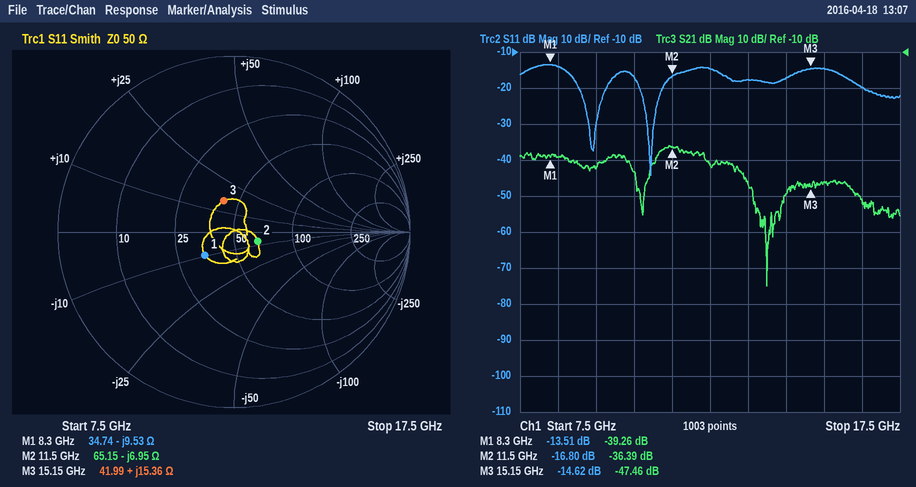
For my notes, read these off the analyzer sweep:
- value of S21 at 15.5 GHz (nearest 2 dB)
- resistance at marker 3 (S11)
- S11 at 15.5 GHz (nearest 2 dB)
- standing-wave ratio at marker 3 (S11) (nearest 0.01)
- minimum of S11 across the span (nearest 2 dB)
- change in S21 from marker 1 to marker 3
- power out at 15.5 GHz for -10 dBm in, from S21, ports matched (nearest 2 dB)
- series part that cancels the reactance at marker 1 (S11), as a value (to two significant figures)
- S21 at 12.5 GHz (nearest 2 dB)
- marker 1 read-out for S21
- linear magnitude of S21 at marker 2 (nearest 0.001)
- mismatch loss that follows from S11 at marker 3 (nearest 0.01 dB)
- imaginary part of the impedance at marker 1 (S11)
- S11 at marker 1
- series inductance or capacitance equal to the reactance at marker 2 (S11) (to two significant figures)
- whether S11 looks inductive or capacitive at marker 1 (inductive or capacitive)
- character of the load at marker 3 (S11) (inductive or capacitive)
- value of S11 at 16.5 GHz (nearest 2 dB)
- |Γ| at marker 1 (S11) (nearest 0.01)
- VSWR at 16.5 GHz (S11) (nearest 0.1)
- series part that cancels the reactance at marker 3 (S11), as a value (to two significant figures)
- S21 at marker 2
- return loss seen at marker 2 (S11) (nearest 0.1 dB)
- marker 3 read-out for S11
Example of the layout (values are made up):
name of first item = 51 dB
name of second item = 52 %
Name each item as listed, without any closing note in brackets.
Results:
value of S21 at 15.5 GHz = -46 dB
resistance at marker 3 = 41.99 Ω
S11 at 15.5 GHz = -14 dB
standing-wave ratio at marker 3 (S11) = 1.46
minimum of S11 across the span = -44 dB
change in S21 from marker 1 to marker 3 = -8.20 dB
power out at 15.5 GHz for -10 dBm in, from S21, ports matched = -56 dBm
series part that cancels the reactance at marker 1 (S11), as a value = 180 pH
S21 at 12.5 GHz = -42 dB
marker 1 read-out for S21 = -39.26 dB
linear magnitude of S21 at marker 2 = 0.015
mismatch loss that follows from S11 at marker 3 = 0.15 dB
imaginary part of the impedance at marker 1 = -9.53 Ω
S11 at marker 1 = -13.51 dB
series inductance or capacitance equal to the reactance at marker 2 (S11) = 2.0 pF
whether S11 looks inductive or capacitive at marker 1 = capacitive
character of the load at marker 3 (S11) = inductive
value of S11 at 16.5 GHz = -20 dB
|Γ| at marker 1 (S11) = 0.21
VSWR at 16.5 GHz (S11) = 1.2
series part that cancels the reactance at marker 3 (S11), as a value = 680 fF
S21 at marker 2 = -36.39 dB
return loss seen at marker 2 (S11) = 16.8 dB
marker 3 read-out for S11 = -14.62 dB
